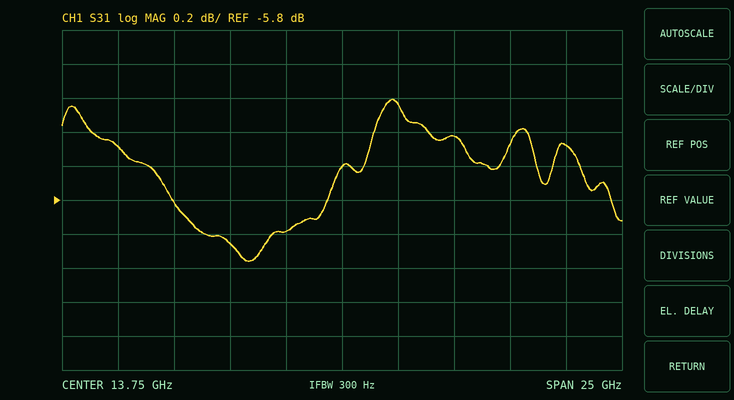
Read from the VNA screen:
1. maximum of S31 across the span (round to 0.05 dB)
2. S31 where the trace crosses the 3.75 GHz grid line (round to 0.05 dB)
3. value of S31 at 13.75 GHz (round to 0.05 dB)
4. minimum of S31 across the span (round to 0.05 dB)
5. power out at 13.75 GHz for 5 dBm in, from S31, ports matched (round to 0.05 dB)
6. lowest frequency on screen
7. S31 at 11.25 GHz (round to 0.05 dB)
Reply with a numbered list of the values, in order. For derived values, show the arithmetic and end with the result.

1. -5.20 dB
2. -5.50 dB
3. -5.60 dB
4. -6.15 dB
5. 5 dBm + (-5.60 dB) = -0.60 dBm
6. 1.25 GHz
7. -6.00 dB
